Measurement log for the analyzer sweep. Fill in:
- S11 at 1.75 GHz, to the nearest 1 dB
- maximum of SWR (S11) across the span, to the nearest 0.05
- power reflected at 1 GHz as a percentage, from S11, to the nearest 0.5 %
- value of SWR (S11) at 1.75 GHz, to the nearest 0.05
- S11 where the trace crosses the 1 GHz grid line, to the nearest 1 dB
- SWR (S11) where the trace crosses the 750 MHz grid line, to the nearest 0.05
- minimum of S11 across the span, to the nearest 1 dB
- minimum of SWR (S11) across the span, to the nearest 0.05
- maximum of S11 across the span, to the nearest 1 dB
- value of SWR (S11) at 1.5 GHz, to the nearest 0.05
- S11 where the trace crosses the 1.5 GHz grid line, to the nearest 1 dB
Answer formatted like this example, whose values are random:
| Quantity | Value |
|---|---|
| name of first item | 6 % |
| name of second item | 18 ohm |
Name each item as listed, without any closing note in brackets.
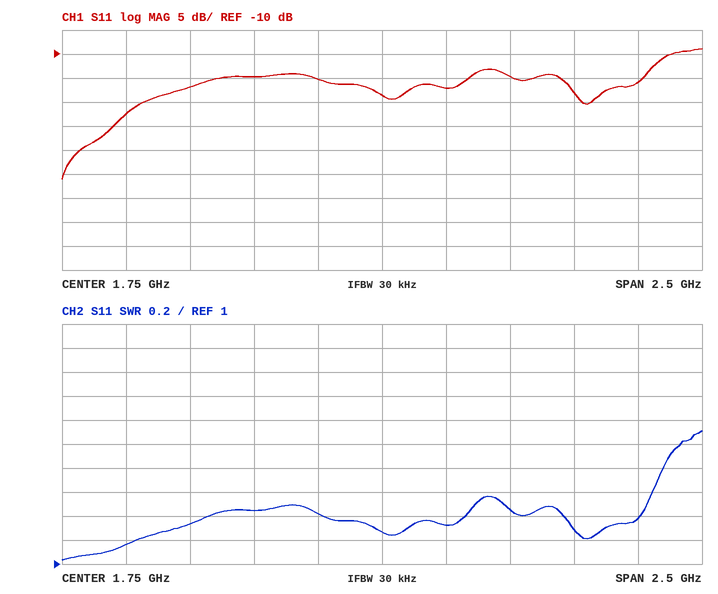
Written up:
| Quantity | Value |
|---|---|
| S11 at 1.75 GHz, to the nearest 1 dB | -19 dB |
| maximum of SWR (S11) across the span, to the nearest 0.05 | 2.10 |
| power reflected at 1 GHz as a percentage, from S11, to the nearest 0.5 % | 2.0 % |
| value of SWR (S11) at 1.75 GHz, to the nearest 0.05 | 1.25 |
| S11 where the trace crosses the 1 GHz grid line, to the nearest 1 dB | -17 dB |
| SWR (S11) where the trace crosses the 750 MHz grid line, to the nearest 0.05 | 1.15 |
| minimum of S11 across the span, to the nearest 1 dB | -36 dB |
| minimum of SWR (S11) across the span, to the nearest 0.05 | 1.05 |
| maximum of S11 across the span, to the nearest 1 dB | -9 dB |
| value of SWR (S11) at 1.5 GHz, to the nearest 0.05 | 1.40 |
| S11 where the trace crosses the 1.5 GHz grid line, to the nearest 1 dB | -15 dB |
